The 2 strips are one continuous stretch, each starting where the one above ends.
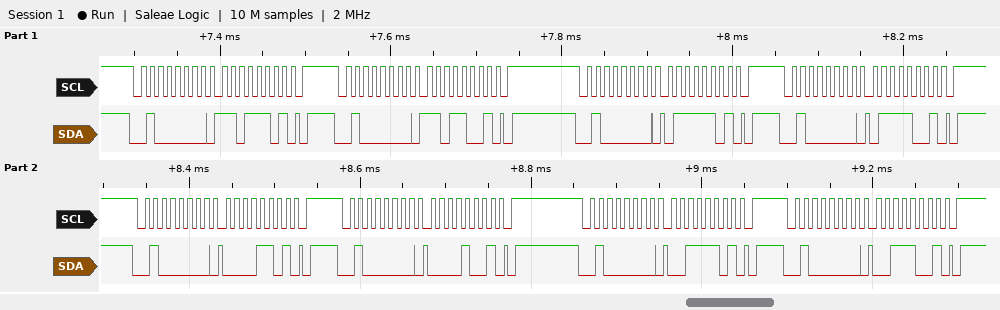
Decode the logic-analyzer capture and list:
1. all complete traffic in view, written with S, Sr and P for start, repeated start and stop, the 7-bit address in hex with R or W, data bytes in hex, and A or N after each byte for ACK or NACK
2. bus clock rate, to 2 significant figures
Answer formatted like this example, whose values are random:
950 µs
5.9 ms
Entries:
S 20W A DD A P S 20W A D9 A P S 20W A 7D A P S 20W A 79 A P S 20W A 0D A P S 20W A 09 A P S 20W A 3D A P S 20W A 39 A P
100 kHz
